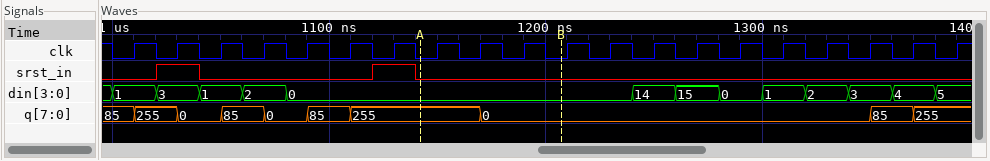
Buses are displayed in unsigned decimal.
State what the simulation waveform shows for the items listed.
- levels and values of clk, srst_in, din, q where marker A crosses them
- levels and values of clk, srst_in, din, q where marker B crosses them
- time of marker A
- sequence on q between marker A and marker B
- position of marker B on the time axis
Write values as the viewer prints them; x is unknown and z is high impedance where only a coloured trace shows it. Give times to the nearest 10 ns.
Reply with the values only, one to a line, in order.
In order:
clk=0, srst_in=0, din=0, q=255
clk=0, srst_in=0, din=0, q=0
1140 ns
255, 0
1210 ns
